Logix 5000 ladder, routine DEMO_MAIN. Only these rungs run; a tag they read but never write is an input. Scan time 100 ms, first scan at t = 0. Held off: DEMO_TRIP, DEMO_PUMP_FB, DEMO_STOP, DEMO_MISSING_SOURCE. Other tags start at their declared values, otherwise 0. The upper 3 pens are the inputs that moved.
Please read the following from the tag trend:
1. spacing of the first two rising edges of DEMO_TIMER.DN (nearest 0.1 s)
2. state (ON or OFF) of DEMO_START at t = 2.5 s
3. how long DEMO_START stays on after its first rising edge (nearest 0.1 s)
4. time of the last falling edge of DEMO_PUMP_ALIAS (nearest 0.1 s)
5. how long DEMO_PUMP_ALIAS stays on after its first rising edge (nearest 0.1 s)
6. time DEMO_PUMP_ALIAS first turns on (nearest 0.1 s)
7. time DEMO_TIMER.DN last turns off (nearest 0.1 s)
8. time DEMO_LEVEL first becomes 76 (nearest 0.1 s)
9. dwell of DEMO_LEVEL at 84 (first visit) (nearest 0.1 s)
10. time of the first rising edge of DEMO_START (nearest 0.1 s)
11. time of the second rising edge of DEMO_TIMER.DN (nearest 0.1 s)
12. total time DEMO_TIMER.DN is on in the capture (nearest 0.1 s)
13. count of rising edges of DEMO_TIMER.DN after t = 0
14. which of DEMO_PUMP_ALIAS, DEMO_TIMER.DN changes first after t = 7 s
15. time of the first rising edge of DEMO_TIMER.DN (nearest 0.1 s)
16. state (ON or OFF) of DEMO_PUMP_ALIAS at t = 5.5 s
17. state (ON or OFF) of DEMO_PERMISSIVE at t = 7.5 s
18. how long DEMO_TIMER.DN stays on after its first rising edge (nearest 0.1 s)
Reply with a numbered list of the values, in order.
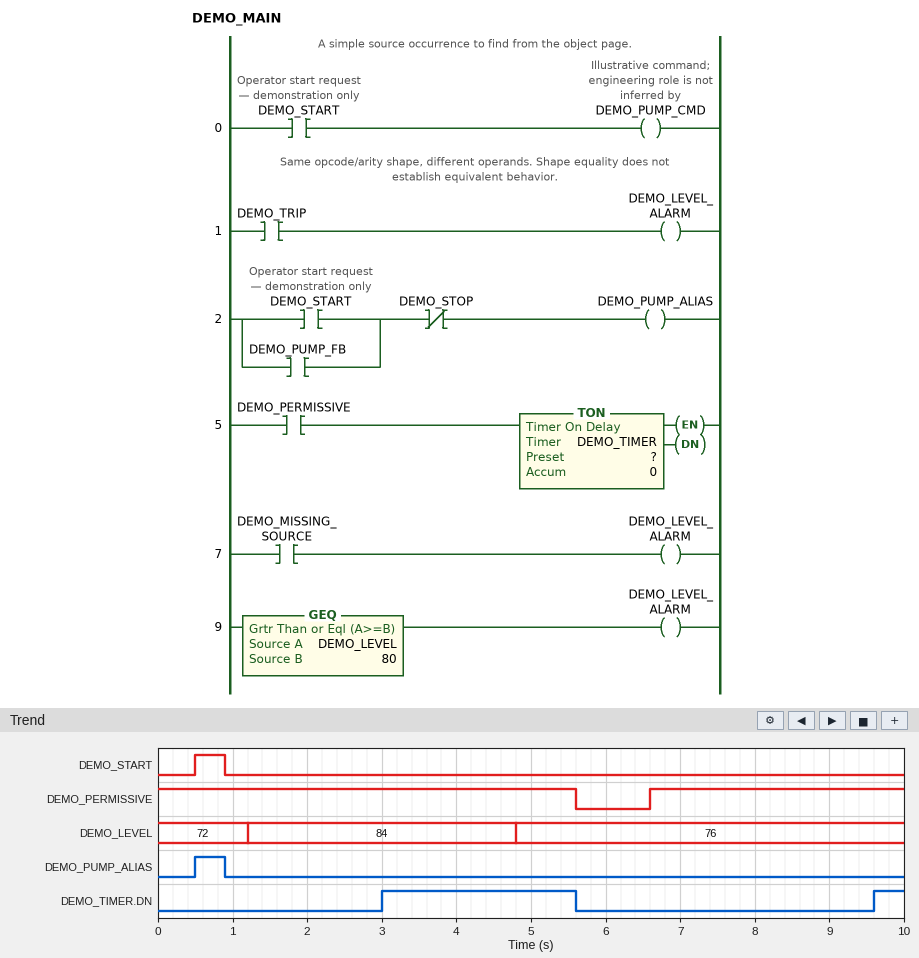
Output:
1. 6.6 s
2. OFF
3. 0.4 s
4. 0.9 s
5. 0.4 s
6. 0.5 s
7. 5.6 s
8. 4.8 s
9. 3.6 s
10. 0.5 s
11. 9.6 s
12. 3.0 s
13. 2
14. DEMO_TIMER.DN
15. 3.0 s
16. OFF
17. ON
18. 2.6 s
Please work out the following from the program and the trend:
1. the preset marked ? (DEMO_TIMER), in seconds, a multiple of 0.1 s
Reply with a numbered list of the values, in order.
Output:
1. 3.0 s
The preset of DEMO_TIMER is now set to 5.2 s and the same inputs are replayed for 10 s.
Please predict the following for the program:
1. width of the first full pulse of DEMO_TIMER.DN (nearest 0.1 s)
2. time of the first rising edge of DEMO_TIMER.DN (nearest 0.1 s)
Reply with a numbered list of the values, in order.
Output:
1. 0.4 s
2. 5.2 s
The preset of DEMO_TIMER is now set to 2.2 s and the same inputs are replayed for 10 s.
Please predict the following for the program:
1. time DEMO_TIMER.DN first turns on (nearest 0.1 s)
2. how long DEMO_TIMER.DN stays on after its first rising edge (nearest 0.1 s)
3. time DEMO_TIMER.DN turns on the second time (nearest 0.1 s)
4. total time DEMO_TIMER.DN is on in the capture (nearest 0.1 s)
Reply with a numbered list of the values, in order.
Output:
1. 2.2 s
2. 3.4 s
3. 8.8 s
4. 4.6 s
